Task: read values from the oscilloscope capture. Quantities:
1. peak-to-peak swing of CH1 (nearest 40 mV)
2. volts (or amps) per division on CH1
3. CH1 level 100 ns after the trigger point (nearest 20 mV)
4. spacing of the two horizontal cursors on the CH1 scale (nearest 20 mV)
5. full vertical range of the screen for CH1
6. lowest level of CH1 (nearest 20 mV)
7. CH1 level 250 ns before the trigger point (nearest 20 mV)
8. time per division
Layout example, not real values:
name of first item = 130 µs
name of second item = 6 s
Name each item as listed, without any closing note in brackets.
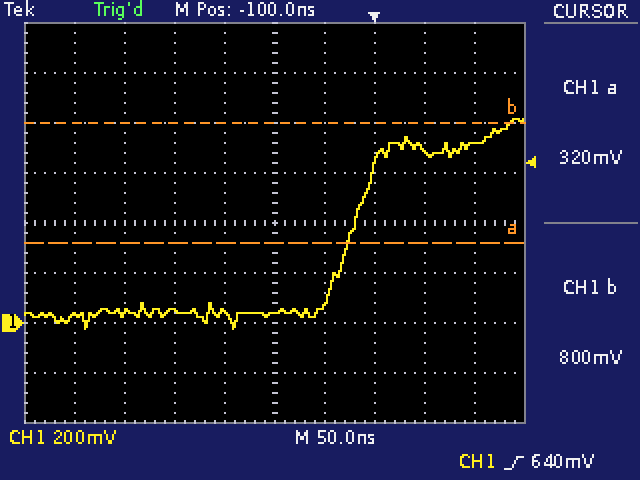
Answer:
peak-to-peak swing of CH1 = 840 mV
volts (or amps) per division on CH1 = 200 mV
CH1 level 100 ns after the trigger point = 720 mV
spacing of the two horizontal cursors on the CH1 scale = 480 mV
full vertical range of the screen for CH1 = 1.6 V
lowest level of CH1 = -20 mV
CH1 level 250 ns before the trigger point = 40 mV
time per division = 50 ns
